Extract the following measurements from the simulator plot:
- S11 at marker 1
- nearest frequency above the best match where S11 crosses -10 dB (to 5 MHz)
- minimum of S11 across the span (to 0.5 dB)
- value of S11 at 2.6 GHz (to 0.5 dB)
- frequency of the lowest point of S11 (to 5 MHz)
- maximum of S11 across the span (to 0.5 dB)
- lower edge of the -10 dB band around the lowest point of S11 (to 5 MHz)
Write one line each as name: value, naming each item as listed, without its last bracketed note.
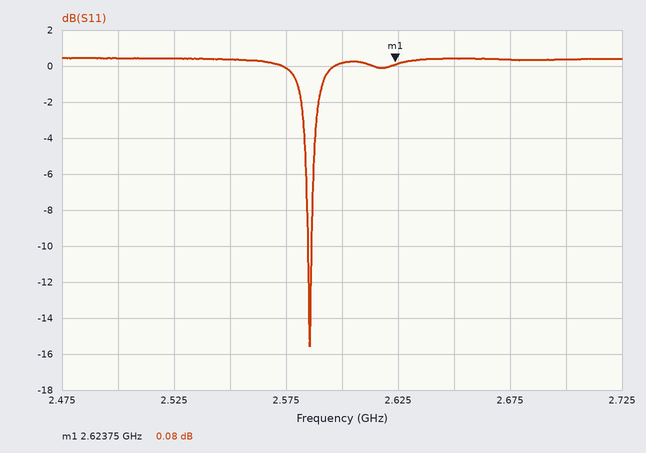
S11 at marker 1: 0.08 dB
nearest frequency above the best match where S11 crosses -10 dB: 2.585 GHz
minimum of S11 across the span: -15.5 dB
value of S11 at 2.6 GHz: 0.0 dB
frequency of the lowest point of S11: 2.585 GHz
maximum of S11 across the span: 0.5 dB
lower edge of the -10 dB band around the lowest point of S11: 2.585 GHz
